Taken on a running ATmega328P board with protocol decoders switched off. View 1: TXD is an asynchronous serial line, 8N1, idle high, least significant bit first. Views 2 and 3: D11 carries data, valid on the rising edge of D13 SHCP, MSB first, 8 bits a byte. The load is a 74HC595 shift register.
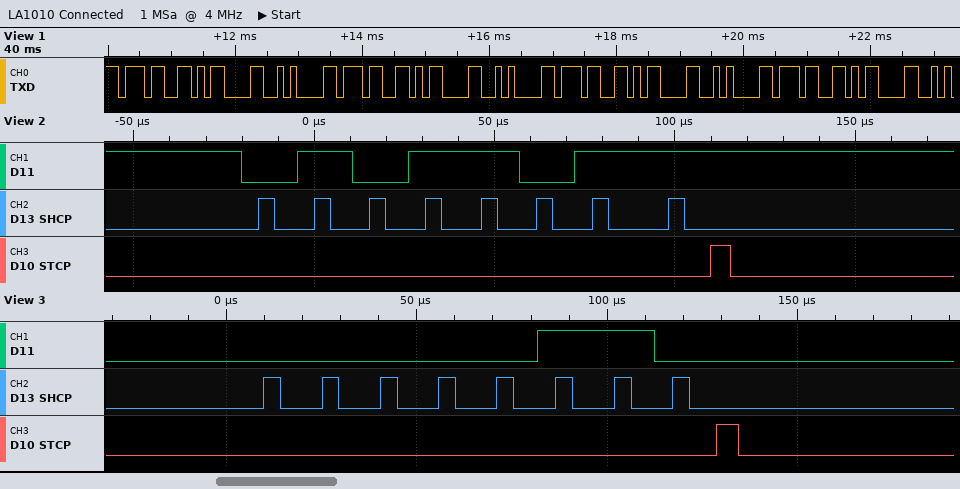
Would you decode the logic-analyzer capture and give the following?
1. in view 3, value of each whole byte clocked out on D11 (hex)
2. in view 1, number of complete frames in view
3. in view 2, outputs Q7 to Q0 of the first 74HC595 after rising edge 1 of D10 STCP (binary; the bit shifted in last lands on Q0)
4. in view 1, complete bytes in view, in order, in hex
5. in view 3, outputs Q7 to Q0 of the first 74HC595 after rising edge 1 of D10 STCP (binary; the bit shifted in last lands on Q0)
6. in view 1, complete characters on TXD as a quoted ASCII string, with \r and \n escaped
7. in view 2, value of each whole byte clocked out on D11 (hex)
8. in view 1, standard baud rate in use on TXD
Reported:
0x06
11
01011011
37 0D 0A 37 0D 0A 37 0D 0A 37 0D
00000110
"7\r\n7\r\n7\r\n7\r"
5B
9600 baud
